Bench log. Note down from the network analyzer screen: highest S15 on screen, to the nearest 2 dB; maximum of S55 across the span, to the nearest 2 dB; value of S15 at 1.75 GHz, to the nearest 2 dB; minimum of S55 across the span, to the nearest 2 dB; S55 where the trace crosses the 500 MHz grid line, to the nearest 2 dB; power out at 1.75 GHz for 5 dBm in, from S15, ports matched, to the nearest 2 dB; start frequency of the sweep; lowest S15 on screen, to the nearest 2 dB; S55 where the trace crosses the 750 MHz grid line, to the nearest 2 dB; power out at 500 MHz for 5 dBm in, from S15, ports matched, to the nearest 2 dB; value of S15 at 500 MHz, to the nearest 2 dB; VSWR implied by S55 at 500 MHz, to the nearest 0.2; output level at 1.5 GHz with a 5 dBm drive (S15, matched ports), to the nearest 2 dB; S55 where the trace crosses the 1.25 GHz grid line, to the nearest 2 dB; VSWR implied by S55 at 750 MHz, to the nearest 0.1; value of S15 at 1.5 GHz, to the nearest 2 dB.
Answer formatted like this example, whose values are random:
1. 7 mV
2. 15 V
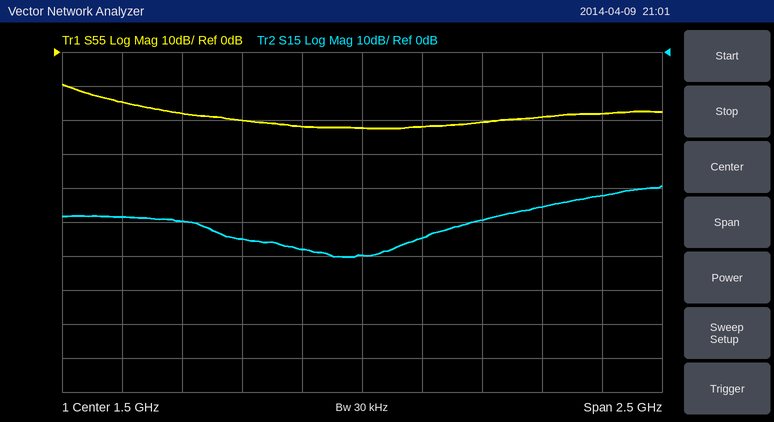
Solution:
1. -40 dB
2. -10 dB
3. -54 dB
4. -22 dB
5. -14 dB
6. -50 dBm
7. 250 MHz
8. -60 dB
9. -18 dB
10. -44 dBm
11. -48 dB
12. 1.4
13. -54 dBm
14. -22 dB
15. 1.3
16. -60 dB
